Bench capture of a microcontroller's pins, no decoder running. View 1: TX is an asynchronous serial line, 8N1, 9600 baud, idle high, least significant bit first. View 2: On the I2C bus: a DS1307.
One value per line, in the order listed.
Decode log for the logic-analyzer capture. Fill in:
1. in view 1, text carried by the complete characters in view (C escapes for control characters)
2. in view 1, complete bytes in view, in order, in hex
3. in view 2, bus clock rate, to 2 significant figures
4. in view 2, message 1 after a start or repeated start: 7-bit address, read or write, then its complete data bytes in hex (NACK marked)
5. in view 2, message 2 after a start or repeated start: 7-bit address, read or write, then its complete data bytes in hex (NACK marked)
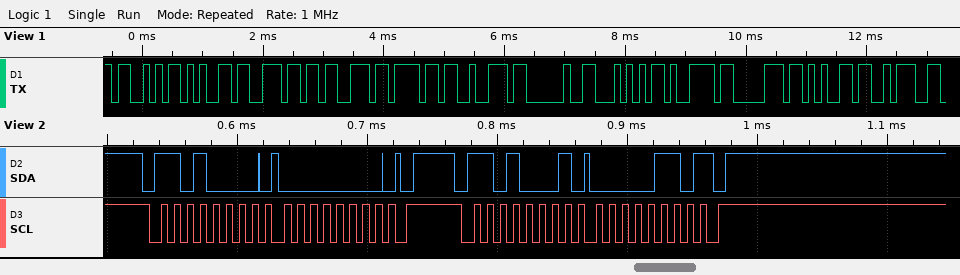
"Sensor Type:"
53 65 6E 73 6F 72 20 54 79 70 65 3A
100 kHz
0x68 write: 00
0x68 read: 06 NACK
